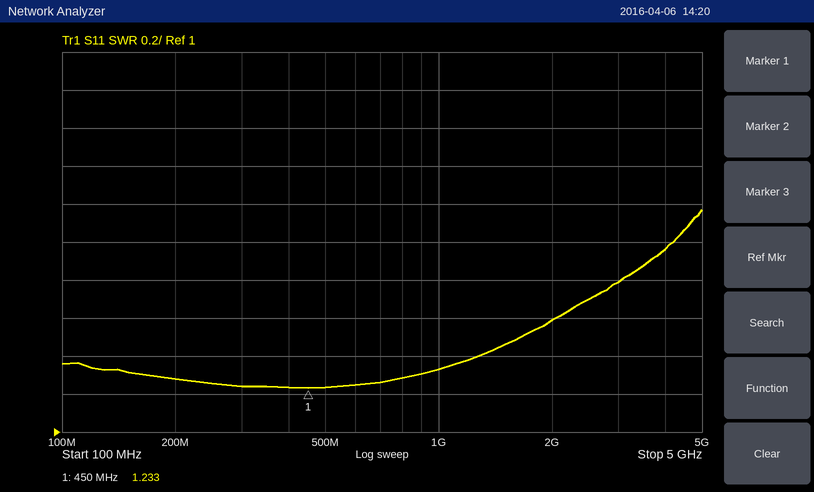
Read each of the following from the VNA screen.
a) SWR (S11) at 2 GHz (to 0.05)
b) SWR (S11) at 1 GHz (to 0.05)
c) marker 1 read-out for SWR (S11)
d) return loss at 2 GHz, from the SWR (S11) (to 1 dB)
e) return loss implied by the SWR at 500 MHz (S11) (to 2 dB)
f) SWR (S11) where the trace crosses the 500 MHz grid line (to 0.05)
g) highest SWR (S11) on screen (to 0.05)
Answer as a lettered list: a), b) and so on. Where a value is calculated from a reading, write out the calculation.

a) 1.60
b) 1.35
c) 1.233
d) −20 log10((1.6 − 1)/(1.6 + 1)) ≈ 13 dB
e) −20 log10((1.25 − 1)/(1.25 + 1)) ≈ 19.1 dB, so 20 dB to the nearest 2 dB
f) 1.25
g) 2.15
